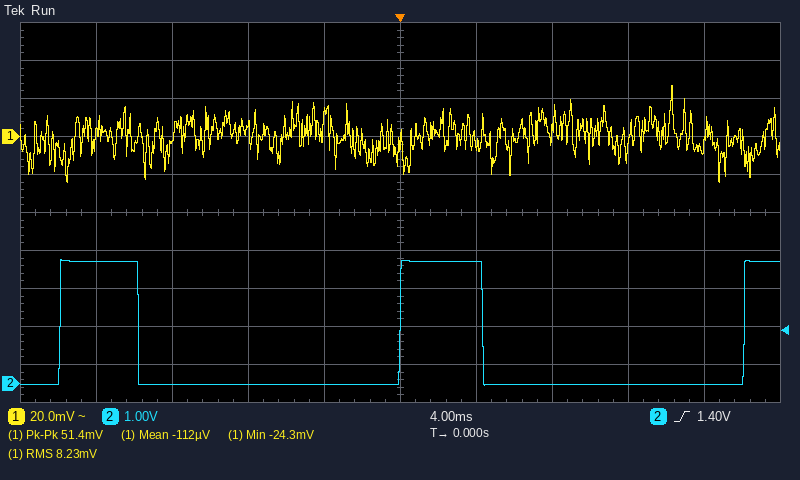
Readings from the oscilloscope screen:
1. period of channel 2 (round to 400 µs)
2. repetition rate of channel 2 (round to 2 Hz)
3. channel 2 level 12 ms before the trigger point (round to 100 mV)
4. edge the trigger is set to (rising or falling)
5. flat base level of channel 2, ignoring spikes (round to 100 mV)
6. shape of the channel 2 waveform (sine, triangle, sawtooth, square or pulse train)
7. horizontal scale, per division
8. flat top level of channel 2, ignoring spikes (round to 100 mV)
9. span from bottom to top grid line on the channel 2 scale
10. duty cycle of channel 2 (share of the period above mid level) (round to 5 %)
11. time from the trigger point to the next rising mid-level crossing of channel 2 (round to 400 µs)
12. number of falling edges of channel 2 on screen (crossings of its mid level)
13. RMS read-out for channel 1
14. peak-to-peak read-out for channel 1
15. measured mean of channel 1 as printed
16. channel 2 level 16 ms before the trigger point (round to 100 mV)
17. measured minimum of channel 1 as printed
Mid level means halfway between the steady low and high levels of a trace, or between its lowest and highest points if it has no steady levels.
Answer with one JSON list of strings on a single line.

["18.0 ms", "56 Hz", "0.0 V", "rising", "0.0 V", "pulse train", "4 ms", "3.2 V", "10 V", "25 %", "18.0 ms", "2", "8.23 mV", "51.4 mV", "-112 µV", "3.2 V", "-24.3 mV"]
